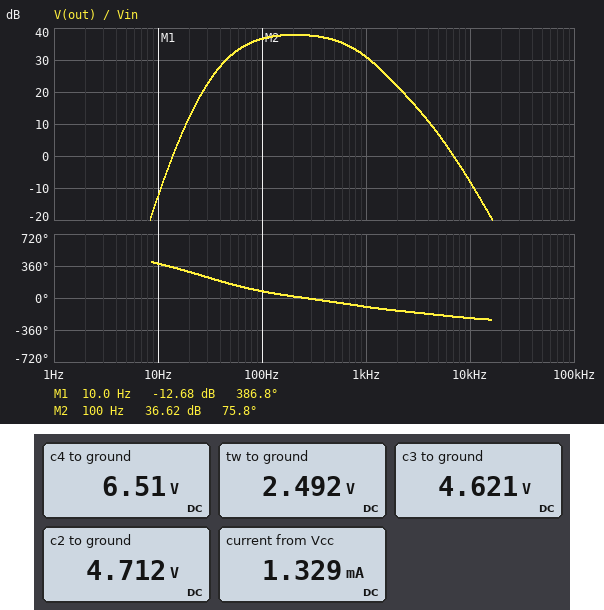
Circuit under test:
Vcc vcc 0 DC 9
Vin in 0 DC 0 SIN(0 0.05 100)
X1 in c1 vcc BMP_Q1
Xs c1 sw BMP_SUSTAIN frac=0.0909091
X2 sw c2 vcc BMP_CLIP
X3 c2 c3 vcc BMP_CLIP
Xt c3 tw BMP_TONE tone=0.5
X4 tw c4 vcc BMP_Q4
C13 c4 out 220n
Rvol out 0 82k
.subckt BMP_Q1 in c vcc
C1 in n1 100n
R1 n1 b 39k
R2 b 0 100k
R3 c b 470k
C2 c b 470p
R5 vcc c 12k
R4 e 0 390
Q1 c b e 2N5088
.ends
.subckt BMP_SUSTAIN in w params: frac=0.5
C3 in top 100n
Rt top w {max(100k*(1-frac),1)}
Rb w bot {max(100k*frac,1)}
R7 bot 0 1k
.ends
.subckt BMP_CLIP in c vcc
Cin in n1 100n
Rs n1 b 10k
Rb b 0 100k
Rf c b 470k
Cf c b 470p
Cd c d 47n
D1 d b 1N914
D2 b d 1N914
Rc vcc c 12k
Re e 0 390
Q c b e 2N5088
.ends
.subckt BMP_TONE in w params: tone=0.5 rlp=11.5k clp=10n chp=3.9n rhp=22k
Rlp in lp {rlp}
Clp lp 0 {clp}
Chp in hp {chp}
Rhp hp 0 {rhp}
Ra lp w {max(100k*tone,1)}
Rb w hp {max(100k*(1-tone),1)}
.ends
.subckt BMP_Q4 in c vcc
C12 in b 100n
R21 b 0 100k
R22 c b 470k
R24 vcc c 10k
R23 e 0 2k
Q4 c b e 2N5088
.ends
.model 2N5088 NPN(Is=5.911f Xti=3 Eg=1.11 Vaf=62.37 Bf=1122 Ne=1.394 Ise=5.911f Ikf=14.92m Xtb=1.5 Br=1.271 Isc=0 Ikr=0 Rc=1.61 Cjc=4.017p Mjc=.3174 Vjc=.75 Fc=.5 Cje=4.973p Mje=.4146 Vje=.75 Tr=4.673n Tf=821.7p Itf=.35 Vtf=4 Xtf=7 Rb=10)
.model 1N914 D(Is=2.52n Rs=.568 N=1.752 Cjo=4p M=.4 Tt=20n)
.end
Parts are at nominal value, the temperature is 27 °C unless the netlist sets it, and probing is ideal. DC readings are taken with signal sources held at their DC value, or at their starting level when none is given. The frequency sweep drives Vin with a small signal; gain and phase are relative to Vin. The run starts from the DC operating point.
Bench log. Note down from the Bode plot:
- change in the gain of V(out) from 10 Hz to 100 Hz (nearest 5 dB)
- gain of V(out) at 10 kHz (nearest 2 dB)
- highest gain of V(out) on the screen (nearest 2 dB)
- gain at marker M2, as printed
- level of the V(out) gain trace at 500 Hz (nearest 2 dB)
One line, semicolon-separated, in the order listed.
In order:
50 dB; -8 dB; 38 dB; 36.62 dB; 36 dB
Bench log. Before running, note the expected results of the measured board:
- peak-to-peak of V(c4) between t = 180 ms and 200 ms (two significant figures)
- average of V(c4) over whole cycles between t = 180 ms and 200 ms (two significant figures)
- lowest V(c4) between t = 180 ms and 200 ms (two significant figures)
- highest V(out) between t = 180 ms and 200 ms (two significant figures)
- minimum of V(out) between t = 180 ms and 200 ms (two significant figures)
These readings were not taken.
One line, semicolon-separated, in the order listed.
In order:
1.3 V; 6.5 V; 5.9 V; 630 mV; -630 mV
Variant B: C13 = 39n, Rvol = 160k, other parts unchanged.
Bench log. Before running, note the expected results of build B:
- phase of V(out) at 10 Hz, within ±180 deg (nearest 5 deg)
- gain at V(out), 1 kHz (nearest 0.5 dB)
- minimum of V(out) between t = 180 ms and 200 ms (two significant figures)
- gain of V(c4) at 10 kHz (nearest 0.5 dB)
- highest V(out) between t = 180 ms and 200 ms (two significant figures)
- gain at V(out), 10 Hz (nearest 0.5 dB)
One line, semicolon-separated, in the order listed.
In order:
55 deg; 31.5 dB; -620 mV; -7.5 dB; 610 mV; -18.5 dB
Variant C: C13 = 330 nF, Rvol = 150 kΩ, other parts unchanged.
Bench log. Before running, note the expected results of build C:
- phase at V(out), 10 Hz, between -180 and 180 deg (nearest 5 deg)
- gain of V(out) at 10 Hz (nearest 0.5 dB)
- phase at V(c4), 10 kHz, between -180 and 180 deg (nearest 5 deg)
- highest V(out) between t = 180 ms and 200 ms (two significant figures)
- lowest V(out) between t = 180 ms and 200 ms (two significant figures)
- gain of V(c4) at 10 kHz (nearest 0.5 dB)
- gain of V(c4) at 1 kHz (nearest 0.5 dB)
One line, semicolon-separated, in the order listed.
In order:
5 deg; -10.5 dB; 135 deg; 660 mV; -670 mV; -7.5 dB; 31.5 dB
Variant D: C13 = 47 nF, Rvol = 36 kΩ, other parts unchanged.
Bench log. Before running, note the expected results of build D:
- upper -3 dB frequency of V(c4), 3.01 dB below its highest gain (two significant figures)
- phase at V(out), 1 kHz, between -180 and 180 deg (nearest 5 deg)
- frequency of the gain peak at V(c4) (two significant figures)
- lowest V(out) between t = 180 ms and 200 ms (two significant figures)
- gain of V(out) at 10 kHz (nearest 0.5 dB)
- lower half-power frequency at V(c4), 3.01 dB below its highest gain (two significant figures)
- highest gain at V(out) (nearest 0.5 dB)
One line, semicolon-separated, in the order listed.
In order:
610 Hz; -95 deg; 180 Hz; -450 mV; -9.0 dB; 64 Hz; 36.5 dB
